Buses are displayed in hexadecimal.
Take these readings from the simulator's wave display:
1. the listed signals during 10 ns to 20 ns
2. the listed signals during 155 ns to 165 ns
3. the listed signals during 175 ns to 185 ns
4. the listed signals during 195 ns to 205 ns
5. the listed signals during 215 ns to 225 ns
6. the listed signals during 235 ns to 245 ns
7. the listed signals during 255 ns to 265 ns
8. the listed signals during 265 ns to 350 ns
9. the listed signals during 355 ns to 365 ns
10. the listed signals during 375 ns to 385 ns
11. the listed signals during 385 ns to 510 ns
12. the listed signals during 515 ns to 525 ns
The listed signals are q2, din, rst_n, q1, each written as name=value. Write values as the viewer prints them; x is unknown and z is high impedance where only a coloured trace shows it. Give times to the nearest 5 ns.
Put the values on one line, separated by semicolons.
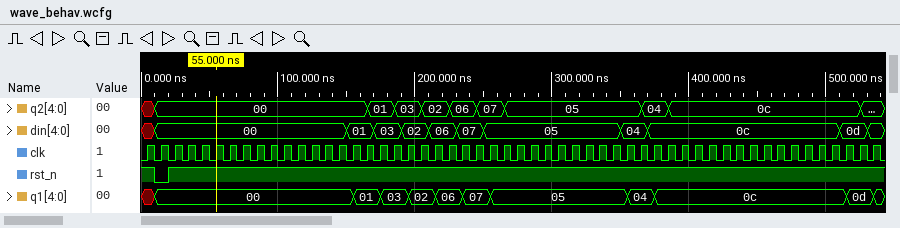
q2=00, din=00, rst_n=0, q1=00; q2=00, din=01, rst_n=1, q1=01; q2=01, din=03, rst_n=1, q1=03; q2=03, din=02, rst_n=1, q1=02; q2=02, din=06, rst_n=1, q1=06; q2=06, din=07, rst_n=1, q1=07; q2=07, din=05, rst_n=1, q1=05; q2=05, din=05, rst_n=1, q1=05; q2=05, din=04, rst_n=1, q1=04; q2=04, din=0c, rst_n=1, q1=0c; q2=0c, din=0c, rst_n=1, q1=0c; q2=0c, din=0d, rst_n=1, q1=0d
